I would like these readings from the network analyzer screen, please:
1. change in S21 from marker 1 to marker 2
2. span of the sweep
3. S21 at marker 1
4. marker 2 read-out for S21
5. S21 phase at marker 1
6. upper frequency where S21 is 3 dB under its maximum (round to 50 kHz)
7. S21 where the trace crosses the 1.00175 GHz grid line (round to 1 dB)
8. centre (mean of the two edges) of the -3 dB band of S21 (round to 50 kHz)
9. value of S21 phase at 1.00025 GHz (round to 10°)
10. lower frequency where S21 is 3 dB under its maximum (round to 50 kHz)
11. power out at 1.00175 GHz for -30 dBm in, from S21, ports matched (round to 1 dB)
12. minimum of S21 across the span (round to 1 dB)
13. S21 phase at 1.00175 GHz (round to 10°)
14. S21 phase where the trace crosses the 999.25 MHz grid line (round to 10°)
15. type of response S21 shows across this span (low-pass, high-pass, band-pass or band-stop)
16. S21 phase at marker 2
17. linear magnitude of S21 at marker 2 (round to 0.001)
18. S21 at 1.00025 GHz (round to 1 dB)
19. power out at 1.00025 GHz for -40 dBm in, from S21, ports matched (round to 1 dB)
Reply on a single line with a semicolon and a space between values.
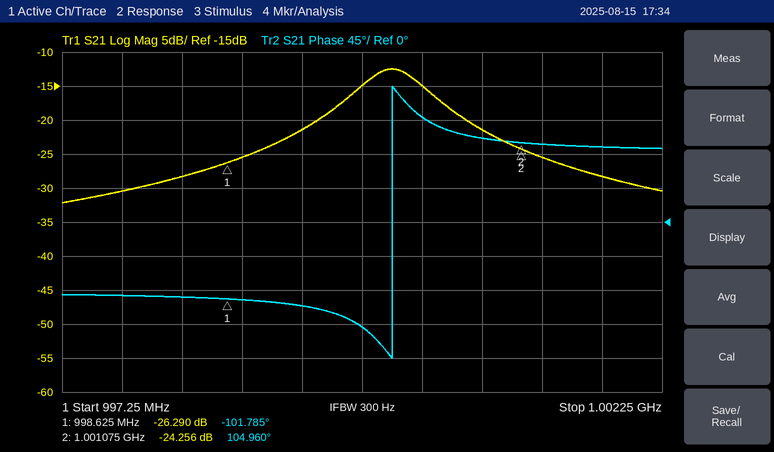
2.034 dB; 5 MHz; -26.290 dB; -24.256 dB; -101.785°; 1.00030 GHz; -28 dB; 1.00000 GHz; 140°; 999.70 MHz; -58 dBm; -32 dB; 100°; -110°; band-pass; 104.960°; 0.061; -15 dB; -55 dBm
